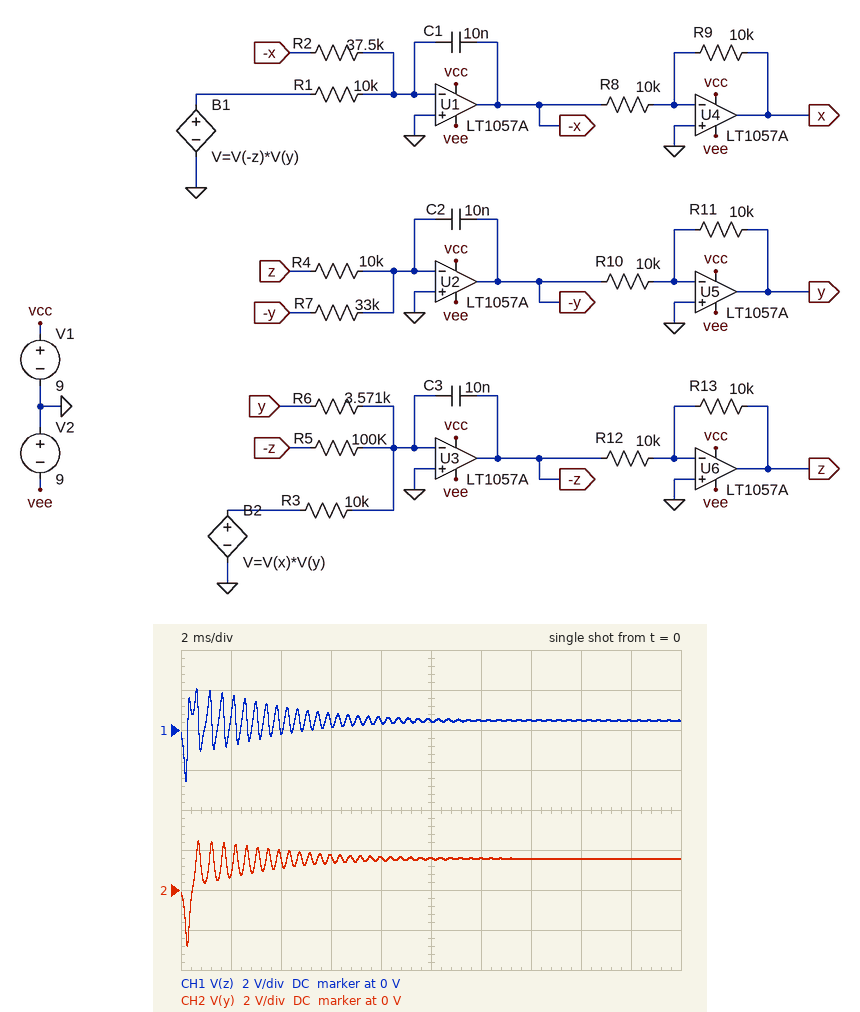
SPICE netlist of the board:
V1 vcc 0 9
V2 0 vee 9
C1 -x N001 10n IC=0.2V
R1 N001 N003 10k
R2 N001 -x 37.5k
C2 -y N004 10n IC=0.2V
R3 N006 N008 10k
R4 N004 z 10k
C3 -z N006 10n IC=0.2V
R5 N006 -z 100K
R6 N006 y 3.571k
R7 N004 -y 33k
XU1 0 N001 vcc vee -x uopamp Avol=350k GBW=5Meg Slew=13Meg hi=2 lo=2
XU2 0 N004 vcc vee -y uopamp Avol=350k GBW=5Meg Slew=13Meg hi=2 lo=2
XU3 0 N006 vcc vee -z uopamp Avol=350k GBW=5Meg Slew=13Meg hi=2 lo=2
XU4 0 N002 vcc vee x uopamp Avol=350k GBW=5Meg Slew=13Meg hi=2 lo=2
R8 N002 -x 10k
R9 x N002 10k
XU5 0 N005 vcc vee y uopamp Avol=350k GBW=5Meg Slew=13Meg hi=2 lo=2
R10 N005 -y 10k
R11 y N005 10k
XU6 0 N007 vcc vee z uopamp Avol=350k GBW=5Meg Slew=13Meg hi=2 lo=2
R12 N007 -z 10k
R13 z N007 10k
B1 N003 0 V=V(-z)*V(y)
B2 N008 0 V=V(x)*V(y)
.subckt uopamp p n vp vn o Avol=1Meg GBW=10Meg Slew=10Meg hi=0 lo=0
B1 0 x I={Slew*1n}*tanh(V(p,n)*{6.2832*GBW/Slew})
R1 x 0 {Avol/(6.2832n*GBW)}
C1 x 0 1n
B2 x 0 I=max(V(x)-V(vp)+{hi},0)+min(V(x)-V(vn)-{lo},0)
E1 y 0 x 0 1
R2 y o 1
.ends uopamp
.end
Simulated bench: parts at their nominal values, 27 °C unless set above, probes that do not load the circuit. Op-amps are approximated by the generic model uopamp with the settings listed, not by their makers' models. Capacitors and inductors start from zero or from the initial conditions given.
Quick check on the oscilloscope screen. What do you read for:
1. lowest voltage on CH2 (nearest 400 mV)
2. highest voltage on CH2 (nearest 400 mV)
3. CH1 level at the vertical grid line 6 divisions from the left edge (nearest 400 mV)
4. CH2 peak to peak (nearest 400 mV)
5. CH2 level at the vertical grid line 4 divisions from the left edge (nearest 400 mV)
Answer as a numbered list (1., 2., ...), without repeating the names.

1. -2.8 V
2. 2.4 V
3. 400 mV
4. 5.2 V
5. 1.6 V
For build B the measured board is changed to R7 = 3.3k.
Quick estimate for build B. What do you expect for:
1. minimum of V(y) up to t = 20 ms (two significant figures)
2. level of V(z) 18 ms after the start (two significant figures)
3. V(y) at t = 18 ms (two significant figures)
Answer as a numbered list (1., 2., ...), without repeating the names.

1. -860 mV
2. -1.4 V
3. -470 mV
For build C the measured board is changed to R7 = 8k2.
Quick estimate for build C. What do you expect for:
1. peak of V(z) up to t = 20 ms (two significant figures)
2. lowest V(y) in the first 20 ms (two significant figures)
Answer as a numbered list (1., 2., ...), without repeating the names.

1. 1.5 V
2. -1.7 V
